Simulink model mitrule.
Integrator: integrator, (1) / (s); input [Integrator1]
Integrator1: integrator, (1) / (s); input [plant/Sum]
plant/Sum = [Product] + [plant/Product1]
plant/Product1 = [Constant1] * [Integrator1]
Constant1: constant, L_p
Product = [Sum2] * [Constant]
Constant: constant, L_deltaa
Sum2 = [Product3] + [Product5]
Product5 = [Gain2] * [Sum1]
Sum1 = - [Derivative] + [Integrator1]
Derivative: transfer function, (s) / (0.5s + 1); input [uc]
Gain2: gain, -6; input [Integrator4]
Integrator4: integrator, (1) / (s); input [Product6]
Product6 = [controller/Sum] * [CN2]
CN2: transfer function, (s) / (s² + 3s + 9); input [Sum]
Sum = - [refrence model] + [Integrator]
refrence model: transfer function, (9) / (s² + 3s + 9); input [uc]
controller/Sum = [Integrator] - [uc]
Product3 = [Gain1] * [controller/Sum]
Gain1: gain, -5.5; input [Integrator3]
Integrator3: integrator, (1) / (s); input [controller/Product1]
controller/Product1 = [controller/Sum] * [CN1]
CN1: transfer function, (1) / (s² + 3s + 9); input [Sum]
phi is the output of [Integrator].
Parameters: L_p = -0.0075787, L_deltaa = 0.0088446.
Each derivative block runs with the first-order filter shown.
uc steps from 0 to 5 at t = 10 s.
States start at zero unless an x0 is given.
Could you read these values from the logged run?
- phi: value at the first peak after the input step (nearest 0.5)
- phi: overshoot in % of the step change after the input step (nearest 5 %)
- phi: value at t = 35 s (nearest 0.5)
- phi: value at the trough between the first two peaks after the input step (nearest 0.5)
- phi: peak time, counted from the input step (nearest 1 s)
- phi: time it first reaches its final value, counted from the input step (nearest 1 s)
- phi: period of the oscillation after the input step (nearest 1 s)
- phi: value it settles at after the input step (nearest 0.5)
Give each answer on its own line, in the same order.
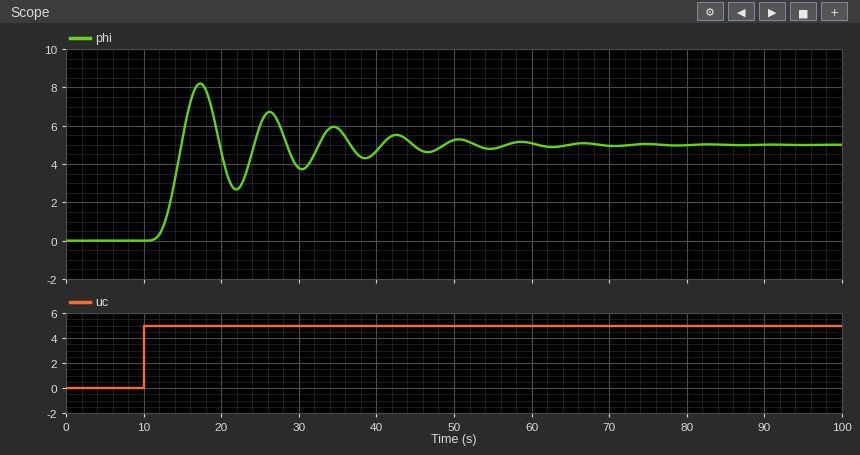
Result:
8.0
65 %
6.0
2.5
7 s
5 s
9 s
5.0
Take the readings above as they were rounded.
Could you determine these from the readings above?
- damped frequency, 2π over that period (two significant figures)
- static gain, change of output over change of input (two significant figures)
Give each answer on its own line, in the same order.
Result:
0.70 rad/s
1.0
